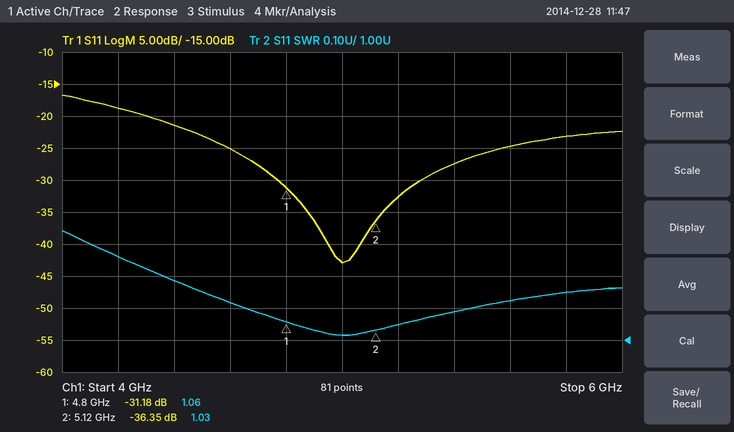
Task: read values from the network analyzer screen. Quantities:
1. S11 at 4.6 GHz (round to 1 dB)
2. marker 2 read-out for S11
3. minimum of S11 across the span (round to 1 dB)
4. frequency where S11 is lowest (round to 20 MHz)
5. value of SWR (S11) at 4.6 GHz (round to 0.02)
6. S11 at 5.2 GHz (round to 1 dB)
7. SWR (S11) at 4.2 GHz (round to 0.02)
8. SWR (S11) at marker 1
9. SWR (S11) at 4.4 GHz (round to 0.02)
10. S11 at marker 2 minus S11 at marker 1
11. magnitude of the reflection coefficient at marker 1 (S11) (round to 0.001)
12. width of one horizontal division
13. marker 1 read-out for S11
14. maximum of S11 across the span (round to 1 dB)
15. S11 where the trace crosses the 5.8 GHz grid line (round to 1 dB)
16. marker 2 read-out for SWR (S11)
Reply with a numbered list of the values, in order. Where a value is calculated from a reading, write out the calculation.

1. -25 dB
2. -36.35 dB
3. -43 dB
4. 5.00 GHz
5. 1.12
6. -33 dB
7. 1.26
8. 1.06
9. 1.18
10. -36.35 − (-31.18) = -5.17 dB
11. 10^(-31.18/20) ≈ 0.028
12. 200 MHz
13. -31.18 dB
14. -17 dB
15. -23 dB
16. 1.03
